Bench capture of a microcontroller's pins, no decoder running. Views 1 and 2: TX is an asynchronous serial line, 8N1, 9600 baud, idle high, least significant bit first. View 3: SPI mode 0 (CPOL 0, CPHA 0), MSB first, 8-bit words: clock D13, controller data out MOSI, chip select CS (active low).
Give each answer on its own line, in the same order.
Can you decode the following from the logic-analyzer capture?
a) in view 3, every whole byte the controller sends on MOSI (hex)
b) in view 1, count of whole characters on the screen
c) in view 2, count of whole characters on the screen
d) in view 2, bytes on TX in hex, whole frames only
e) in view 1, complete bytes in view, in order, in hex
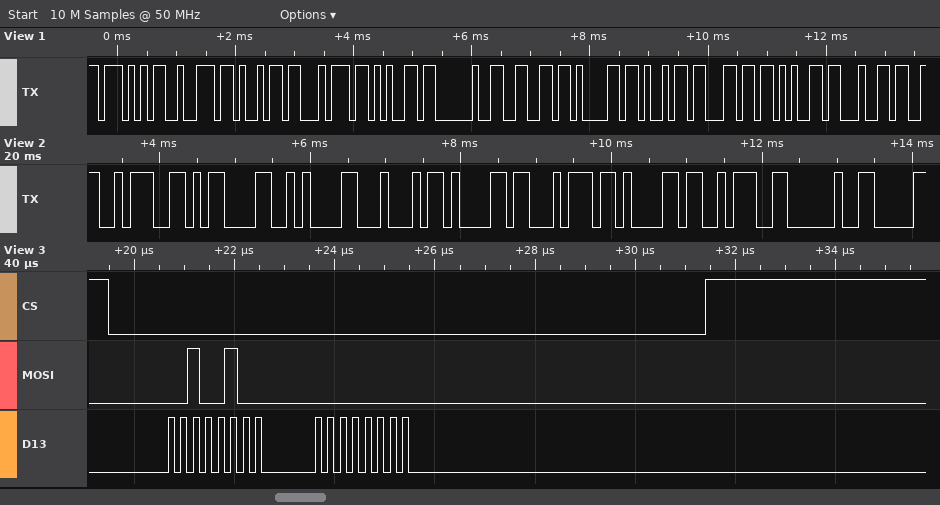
0x24 0x00
12
9
3A 0D 0A 44 61 74 61 3A 20
57 72 69 74 65 20 66 61 69 6C 65 64
